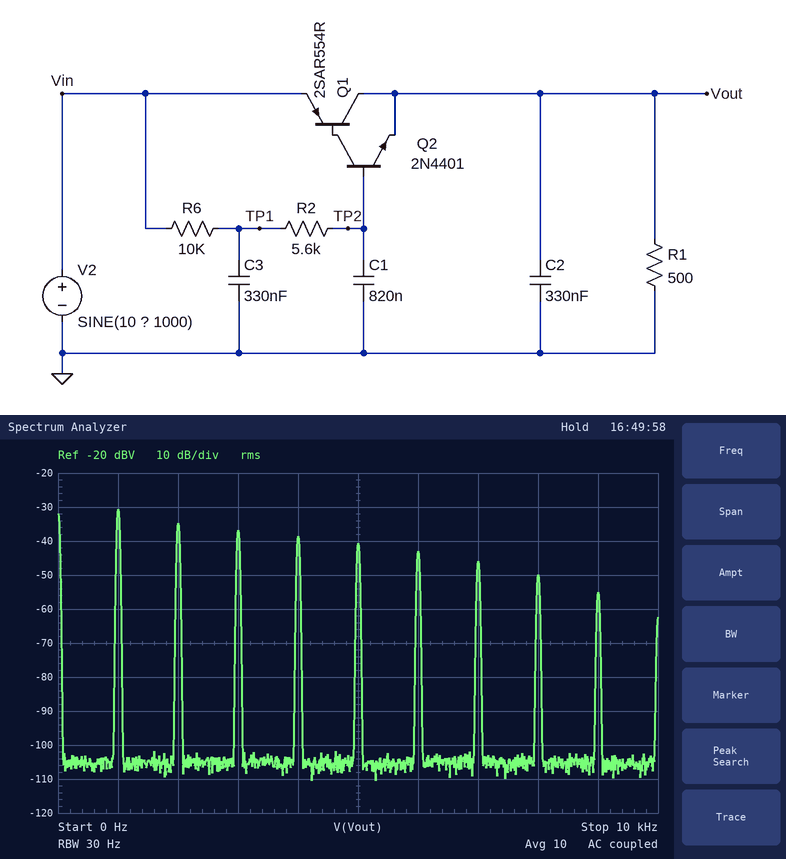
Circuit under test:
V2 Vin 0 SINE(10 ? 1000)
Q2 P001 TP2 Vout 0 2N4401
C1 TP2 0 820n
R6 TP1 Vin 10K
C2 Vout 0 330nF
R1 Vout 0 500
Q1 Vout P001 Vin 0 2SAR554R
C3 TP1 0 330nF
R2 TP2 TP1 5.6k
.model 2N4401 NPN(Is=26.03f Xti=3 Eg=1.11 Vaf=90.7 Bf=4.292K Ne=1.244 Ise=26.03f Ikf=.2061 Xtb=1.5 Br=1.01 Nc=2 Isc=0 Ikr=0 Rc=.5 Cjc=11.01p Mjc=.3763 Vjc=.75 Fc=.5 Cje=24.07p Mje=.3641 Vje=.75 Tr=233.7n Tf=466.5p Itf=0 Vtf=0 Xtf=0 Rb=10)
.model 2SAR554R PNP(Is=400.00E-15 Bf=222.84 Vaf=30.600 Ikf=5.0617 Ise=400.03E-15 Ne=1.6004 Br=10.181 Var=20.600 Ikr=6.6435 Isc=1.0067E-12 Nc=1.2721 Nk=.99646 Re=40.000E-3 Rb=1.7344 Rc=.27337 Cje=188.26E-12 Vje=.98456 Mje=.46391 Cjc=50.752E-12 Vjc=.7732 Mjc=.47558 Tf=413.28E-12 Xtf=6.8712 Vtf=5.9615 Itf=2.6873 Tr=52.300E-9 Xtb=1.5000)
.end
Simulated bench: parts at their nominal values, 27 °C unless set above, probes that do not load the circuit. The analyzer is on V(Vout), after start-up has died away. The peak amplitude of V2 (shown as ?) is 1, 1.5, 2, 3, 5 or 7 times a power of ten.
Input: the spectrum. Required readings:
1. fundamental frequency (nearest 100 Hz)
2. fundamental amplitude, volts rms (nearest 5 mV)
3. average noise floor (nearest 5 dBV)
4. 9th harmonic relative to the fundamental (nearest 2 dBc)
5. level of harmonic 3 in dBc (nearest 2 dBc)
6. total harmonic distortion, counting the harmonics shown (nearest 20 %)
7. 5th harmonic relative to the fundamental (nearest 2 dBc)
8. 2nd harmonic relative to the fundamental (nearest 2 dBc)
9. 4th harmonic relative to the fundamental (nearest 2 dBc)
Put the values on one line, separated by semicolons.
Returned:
1.0 kHz; 30 mV; -105 dBV; -24 dBc; -6 dBc; 100 %; -10 dBc; -4 dBc; -8 dBc
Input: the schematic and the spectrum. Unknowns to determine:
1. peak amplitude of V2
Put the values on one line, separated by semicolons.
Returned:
1.5 V
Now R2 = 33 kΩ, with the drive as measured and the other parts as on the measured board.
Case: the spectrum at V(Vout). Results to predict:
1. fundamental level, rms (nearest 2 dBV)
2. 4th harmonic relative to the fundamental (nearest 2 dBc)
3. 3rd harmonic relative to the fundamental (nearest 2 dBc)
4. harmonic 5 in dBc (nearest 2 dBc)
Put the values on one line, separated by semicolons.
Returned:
-38 dBV; -6 dBc; -4 dBc; -6 dBc
